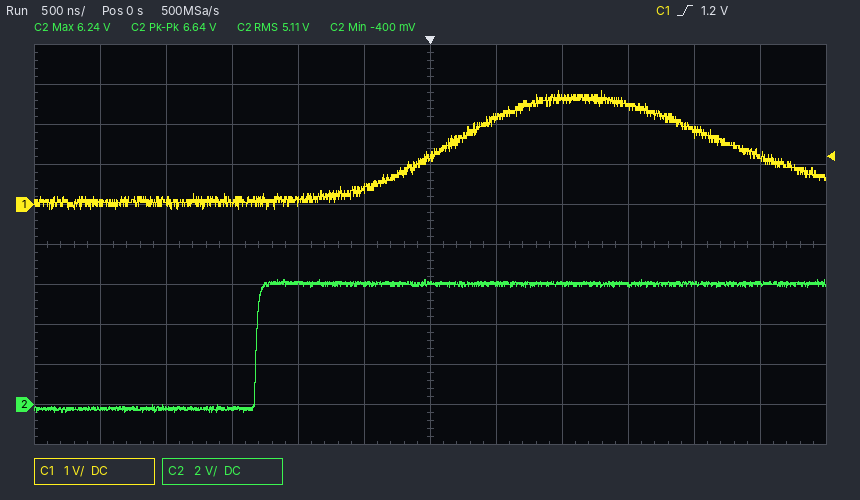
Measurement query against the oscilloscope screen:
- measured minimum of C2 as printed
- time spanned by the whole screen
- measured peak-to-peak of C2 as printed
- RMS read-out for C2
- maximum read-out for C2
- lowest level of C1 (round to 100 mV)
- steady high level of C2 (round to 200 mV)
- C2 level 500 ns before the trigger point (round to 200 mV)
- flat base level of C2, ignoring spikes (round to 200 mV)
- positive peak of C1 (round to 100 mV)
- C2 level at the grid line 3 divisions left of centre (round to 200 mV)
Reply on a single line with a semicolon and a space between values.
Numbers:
-400 mV; 6 µs; 6.64 V; 5.11 V; 6.24 V; -100 mV; 6.0 V; 6.0 V; -200 mV; 2.8 V; -200 mV
